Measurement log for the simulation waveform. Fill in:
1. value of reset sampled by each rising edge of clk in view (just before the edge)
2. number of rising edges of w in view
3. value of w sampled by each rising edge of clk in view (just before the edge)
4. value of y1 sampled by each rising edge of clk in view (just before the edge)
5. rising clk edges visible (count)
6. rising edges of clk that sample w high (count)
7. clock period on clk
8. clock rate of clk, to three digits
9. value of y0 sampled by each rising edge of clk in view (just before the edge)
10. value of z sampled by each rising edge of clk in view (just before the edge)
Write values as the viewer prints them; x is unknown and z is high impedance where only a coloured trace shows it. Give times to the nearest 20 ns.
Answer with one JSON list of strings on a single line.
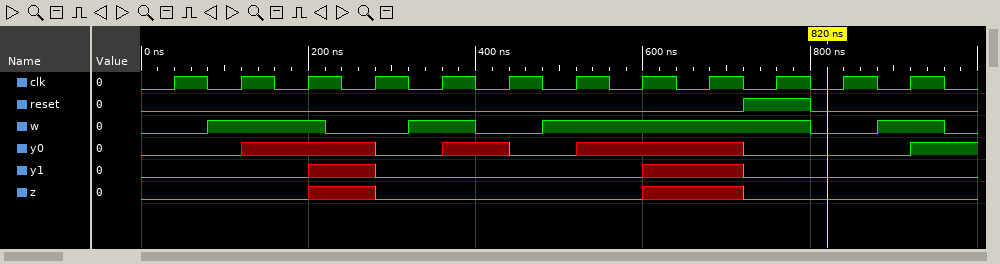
["0 0 0 0 0 0 0 0 0 1 0 0", "4", "0 1 1 0 1 0 1 1 1 1 0 1", "0 0 0 x 0 0 0 0 x 0 0 0", "12", "8", "80 ns", "12.5 MHz", "0 0 x x 0 x 0 x x 0 0 0", "0 0 0 x 0 0 0 0 x 0 0 0"]
